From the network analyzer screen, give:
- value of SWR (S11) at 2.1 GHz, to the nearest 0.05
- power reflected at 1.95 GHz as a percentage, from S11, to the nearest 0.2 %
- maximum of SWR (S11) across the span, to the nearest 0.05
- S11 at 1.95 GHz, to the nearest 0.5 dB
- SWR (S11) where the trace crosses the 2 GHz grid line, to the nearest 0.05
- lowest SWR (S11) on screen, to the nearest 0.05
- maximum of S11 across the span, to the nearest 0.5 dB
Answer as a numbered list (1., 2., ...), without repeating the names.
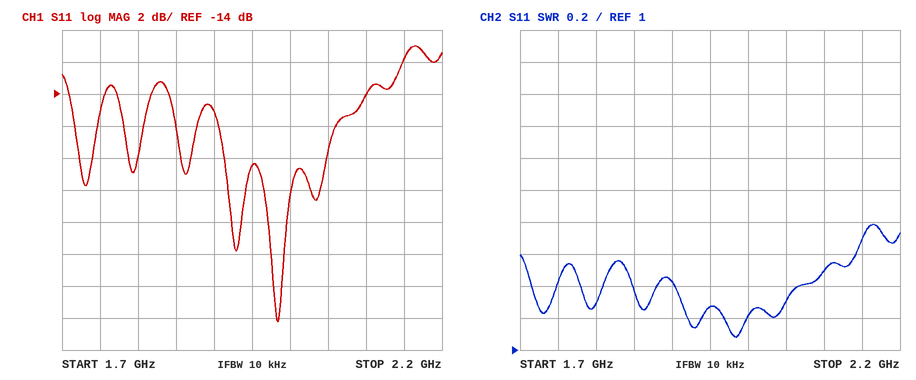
1. 1.50
2. 1.4 %
3. 1.80
4. -18.5 dB
5. 1.20
6. 1.10
7. -11.0 dB
